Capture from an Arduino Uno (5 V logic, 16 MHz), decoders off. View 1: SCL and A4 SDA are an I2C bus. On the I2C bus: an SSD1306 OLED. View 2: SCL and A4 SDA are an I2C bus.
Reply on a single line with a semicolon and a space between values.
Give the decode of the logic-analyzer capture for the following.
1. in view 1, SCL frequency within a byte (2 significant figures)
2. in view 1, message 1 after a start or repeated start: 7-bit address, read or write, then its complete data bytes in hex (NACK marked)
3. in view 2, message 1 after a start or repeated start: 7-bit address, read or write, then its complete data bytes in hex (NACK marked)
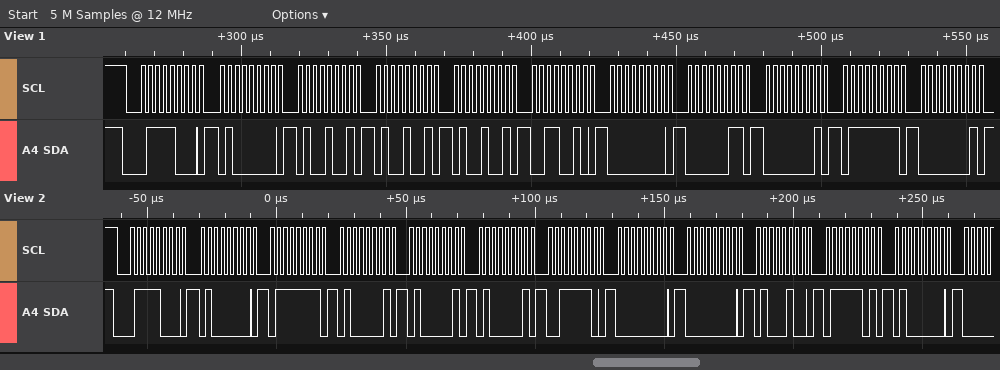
400 kHz; 0x3C write: 40 49 49 49 32 00 03 01 7F 01; 0x3C write: 40 7F 41 41 41 3E 00 00 44 7D 40
